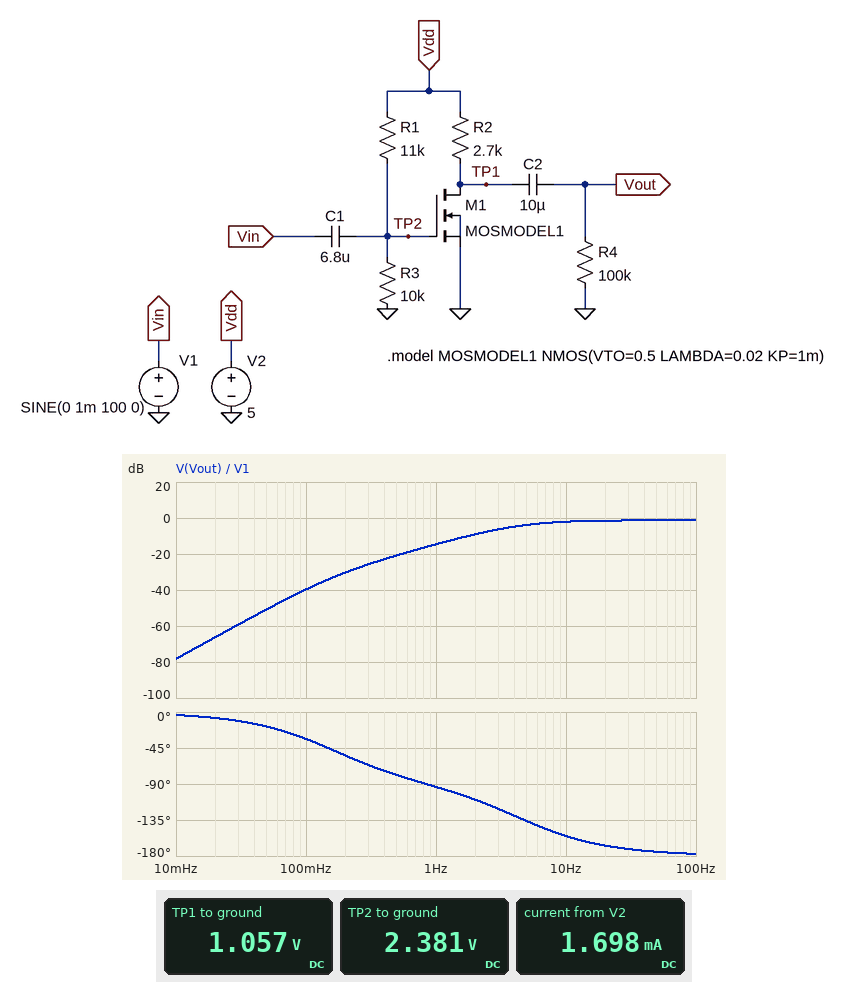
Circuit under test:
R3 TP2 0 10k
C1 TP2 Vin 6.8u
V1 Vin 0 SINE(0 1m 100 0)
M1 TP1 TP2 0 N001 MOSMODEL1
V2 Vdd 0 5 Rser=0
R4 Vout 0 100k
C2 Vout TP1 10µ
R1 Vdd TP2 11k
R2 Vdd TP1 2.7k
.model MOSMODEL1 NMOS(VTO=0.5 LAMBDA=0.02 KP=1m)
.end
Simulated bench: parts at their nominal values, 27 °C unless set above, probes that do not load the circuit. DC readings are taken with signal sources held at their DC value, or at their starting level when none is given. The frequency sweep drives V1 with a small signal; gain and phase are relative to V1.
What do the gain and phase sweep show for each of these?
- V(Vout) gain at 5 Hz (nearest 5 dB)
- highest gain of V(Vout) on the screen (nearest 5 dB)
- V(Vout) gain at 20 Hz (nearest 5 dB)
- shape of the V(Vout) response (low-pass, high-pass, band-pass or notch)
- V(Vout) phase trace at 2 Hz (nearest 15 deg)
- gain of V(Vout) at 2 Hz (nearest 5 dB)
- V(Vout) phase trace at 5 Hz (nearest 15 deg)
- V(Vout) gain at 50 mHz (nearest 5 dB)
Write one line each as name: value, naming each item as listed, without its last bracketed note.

V(Vout) gain at 5 Hz: -5 dB
highest gain of V(Vout) on the screen: 0 dB
V(Vout) gain at 20 Hz: 0 dB
shape of the V(Vout) response: high-pass
V(Vout) phase trace at 2 Hz: -105 deg
gain of V(Vout) at 2 Hz: -10 dB
V(Vout) phase trace at 5 Hz: -135 deg
V(Vout) gain at 50 mHz: -50 dB
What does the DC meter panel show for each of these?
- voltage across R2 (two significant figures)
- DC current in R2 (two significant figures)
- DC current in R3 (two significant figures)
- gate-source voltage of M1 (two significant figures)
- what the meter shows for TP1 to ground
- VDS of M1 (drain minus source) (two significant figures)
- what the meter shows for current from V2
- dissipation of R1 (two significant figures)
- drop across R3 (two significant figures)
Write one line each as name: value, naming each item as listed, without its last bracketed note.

voltage across R2: 3.9 V
DC current in R2: 1.5 mA
DC current in R3: 240 µA
gate-source voltage of M1: 2.4 V
what the meter shows for TP1 to ground: 1.057 V
VDS of M1 (drain minus source): 1.1 V
what the meter shows for current from V2: 1.698 mA
dissipation of R1: 620 µW
drop across R3: 2.4 V
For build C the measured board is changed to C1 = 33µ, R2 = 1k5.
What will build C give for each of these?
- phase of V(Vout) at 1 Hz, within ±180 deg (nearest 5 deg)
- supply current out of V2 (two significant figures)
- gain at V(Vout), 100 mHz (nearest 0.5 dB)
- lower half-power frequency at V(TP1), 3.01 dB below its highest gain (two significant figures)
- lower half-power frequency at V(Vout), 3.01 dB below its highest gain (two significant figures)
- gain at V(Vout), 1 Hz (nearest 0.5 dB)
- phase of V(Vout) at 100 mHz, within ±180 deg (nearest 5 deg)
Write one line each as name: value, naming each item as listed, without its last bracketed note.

phase of V(Vout) at 1 Hz, within ±180 deg: -130 deg
supply current out of V2: 2.1 mA
gain at V(Vout), 100 mHz: -16.0 dB
lower half-power frequency at V(TP1), 3.01 dB below its highest gain: 920 mHz
lower half-power frequency at V(Vout), 3.01 dB below its highest gain: 950 mHz
gain at V(Vout), 1 Hz: 6.0 dB
phase of V(Vout) at 100 mHz, within ±180 deg: -40 deg
